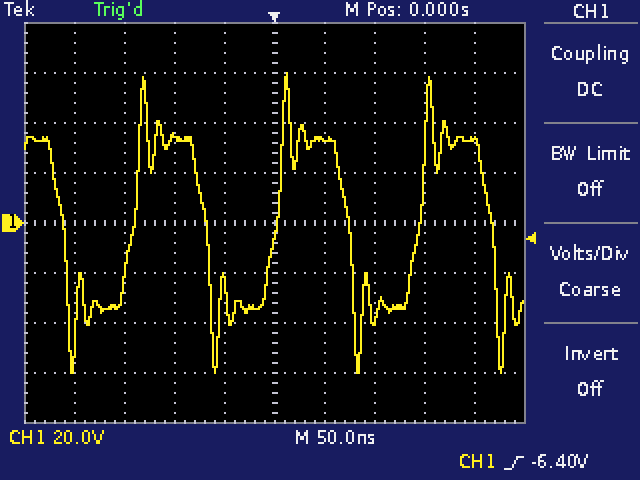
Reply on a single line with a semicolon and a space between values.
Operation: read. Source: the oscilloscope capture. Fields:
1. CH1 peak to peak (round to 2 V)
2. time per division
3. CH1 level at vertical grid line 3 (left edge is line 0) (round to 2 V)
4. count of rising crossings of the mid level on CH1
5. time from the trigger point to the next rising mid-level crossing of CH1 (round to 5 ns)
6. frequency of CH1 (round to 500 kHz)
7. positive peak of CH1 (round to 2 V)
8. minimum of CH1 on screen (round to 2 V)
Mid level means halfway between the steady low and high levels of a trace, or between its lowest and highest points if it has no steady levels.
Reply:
120 V; 50 ns; 34 V; 3; 5 ns; 7.0 MHz; 60 V; -60 V
